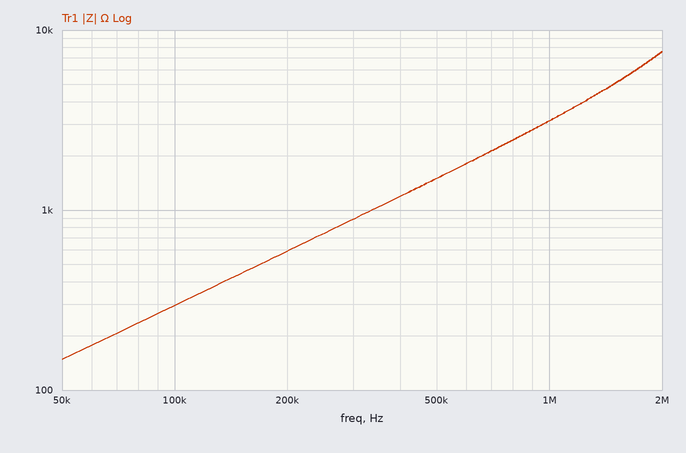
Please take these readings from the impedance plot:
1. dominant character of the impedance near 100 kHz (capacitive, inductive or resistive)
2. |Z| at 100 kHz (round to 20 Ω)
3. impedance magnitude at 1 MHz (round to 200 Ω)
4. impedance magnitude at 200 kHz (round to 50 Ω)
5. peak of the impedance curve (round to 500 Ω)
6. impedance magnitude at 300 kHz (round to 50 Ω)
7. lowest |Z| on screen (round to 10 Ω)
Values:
inductive
300 Ω
3.2 kΩ
600 Ω
7.5 kΩ
900 Ω
150 Ω
